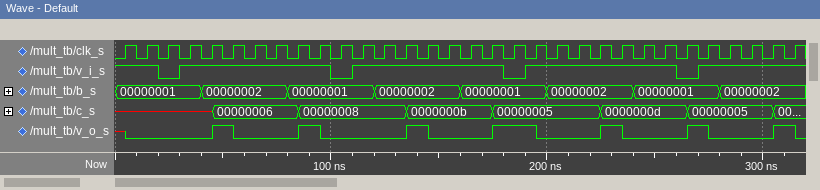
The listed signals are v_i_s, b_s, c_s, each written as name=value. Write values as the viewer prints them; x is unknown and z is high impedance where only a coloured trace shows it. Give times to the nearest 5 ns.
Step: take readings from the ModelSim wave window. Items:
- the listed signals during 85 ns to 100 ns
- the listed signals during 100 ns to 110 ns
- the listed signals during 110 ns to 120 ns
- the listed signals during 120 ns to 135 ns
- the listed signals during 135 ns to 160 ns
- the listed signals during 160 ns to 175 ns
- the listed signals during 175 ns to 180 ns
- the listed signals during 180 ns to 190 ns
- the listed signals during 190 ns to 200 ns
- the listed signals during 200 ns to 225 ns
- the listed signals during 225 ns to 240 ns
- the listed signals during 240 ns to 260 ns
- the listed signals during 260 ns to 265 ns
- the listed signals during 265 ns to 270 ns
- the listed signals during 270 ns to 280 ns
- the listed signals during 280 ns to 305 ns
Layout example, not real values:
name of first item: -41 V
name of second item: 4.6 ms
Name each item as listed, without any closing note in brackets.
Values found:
the listed signals during 85 ns to 100 ns: v_i_s=1, b_s=00000001, c_s=00000008
the listed signals during 100 ns to 110 ns: v_i_s=0, b_s=00000001, c_s=00000008
the listed signals during 110 ns to 120 ns: v_i_s=1, b_s=00000001, c_s=00000008
the listed signals during 120 ns to 135 ns: v_i_s=1, b_s=00000002, c_s=00000008
the listed signals during 135 ns to 160 ns: v_i_s=1, b_s=00000002, c_s=0000000b
the listed signals during 160 ns to 175 ns: v_i_s=1, b_s=00000001, c_s=0000000b
the listed signals during 175 ns to 180 ns: v_i_s=1, b_s=00000001, c_s=00000005
the listed signals during 180 ns to 190 ns: v_i_s=0, b_s=00000001, c_s=00000005
the listed signals during 190 ns to 200 ns: v_i_s=1, b_s=00000001, c_s=00000005
the listed signals during 200 ns to 225 ns: v_i_s=1, b_s=00000002, c_s=00000005
the listed signals during 225 ns to 240 ns: v_i_s=1, b_s=00000002, c_s=0000000d
the listed signals during 240 ns to 260 ns: v_i_s=1, b_s=00000001, c_s=0000000d
the listed signals during 260 ns to 265 ns: v_i_s=0, b_s=00000001, c_s=0000000d
the listed signals during 265 ns to 270 ns: v_i_s=0, b_s=00000001, c_s=00000005
the listed signals during 270 ns to 280 ns: v_i_s=1, b_s=00000001, c_s=00000005
the listed signals during 280 ns to 305 ns: v_i_s=1, b_s=00000002, c_s=00000005
